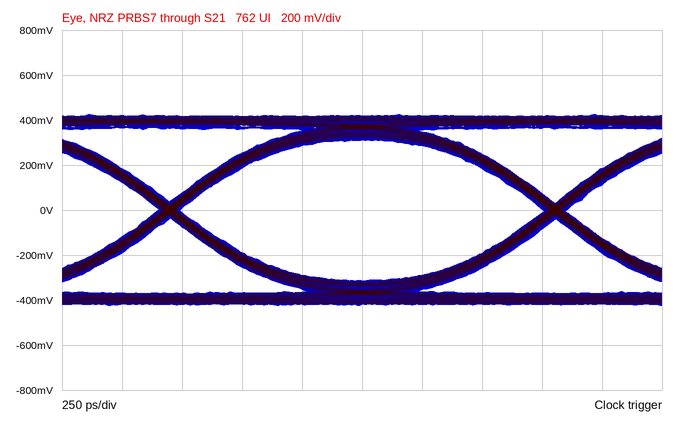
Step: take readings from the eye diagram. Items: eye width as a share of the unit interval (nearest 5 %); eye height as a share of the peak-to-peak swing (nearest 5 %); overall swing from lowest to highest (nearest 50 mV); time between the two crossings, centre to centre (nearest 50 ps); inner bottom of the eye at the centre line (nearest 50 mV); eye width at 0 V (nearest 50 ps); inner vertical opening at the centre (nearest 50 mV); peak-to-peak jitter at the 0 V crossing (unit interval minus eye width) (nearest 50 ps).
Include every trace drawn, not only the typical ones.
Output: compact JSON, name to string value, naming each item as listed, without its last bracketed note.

{"eye width as a share of the unit interval": "95 %", "eye height as a share of the peak-to-peak swing": "75 %", "overall swing from lowest to highest": "850 mV", "time between the two crossings, centre to centre": "1.60 ns", "inner bottom of the eye at the centre line": "-300 mV", "eye width at 0 V": "1.50 ns", "inner vertical opening at the centre": "650 mV", "peak-to-peak jitter at the 0 V crossing (unit interval minus eye width)": "100 ps"}
